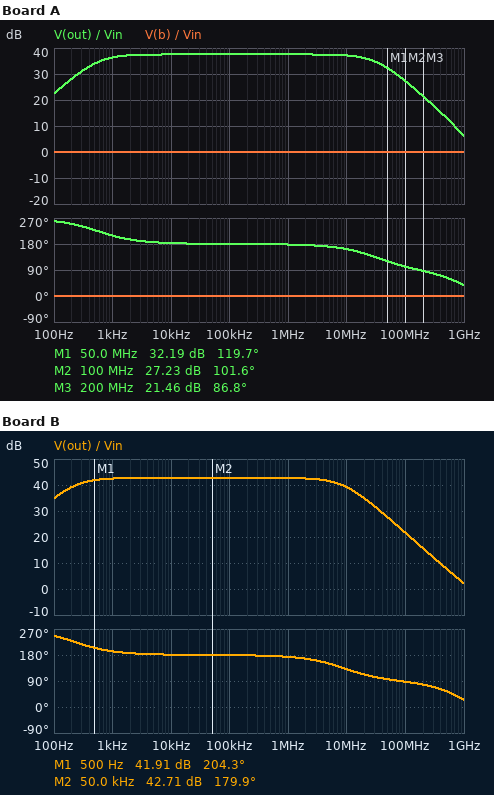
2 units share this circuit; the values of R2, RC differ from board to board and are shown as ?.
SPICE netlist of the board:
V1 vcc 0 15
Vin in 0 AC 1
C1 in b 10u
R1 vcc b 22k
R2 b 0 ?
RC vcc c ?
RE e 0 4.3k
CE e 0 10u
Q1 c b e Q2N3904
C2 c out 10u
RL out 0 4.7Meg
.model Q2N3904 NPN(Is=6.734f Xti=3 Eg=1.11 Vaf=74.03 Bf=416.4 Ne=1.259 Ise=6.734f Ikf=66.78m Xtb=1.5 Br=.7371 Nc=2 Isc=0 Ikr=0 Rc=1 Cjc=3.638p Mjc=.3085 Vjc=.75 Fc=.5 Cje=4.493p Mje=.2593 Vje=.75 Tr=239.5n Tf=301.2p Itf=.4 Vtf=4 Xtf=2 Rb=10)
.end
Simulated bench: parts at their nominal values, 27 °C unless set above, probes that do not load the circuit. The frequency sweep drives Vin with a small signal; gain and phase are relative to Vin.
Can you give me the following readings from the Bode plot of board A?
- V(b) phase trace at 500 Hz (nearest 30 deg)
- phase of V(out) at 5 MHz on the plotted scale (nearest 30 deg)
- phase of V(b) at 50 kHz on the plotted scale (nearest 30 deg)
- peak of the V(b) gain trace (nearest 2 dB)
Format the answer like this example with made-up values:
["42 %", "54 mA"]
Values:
["0 deg", "180 deg", "0 deg", "0 dB"]
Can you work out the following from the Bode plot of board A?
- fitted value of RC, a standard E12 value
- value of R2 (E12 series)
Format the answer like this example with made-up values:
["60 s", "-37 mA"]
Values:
["2.2 kΩ", "10 kΩ"]
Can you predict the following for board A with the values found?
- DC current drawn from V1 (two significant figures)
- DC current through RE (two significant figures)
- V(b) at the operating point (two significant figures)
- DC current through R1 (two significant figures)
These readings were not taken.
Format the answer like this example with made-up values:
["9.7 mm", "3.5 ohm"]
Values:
["1.4 mA", "930 µA", "4.6 V", "470 µA"]
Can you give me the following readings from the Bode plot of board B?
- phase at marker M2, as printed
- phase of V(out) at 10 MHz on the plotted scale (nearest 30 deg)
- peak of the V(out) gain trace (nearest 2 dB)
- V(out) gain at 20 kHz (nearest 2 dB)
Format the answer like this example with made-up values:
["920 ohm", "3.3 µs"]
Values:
["179.9 deg", "120 deg", "42 dB", "42 dB"]
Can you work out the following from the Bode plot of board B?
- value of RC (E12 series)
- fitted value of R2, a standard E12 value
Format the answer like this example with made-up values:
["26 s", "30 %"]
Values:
["10 kΩ", "3.9 kΩ"]
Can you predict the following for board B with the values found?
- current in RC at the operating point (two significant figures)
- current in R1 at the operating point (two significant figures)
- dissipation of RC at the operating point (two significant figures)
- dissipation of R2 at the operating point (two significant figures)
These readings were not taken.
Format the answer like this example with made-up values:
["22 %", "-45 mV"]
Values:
["370 µA", "580 µA", "1.4 mW", "1.3 mW"]
